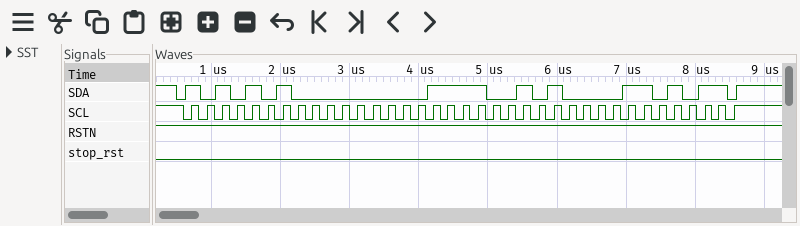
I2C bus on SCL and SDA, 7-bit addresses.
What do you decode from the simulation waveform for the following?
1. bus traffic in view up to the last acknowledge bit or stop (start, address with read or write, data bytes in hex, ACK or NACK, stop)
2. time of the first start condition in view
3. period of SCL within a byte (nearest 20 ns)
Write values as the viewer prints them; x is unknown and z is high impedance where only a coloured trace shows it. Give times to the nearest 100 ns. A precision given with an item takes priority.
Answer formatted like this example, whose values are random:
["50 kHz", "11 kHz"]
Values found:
["start, address 55 write ACK, 01 NACK, CA ACK, 35 NACK, stop", "500 ns", "220 ns"]
